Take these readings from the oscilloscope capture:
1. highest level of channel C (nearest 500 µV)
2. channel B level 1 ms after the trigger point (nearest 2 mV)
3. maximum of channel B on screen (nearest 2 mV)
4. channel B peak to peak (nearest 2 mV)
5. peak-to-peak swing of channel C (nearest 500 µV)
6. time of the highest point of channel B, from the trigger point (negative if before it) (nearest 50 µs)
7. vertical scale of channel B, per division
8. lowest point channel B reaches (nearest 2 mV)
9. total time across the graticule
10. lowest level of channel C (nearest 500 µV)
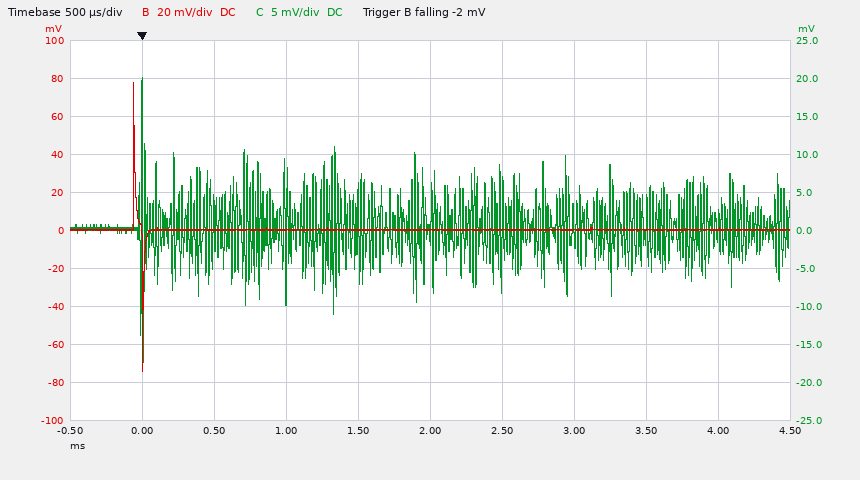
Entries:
20.0 mV
0 mV
78 mV
152 mV
37.5 mV
-50 µs
20 mV
-74 mV
5 ms
-17.5 mV
